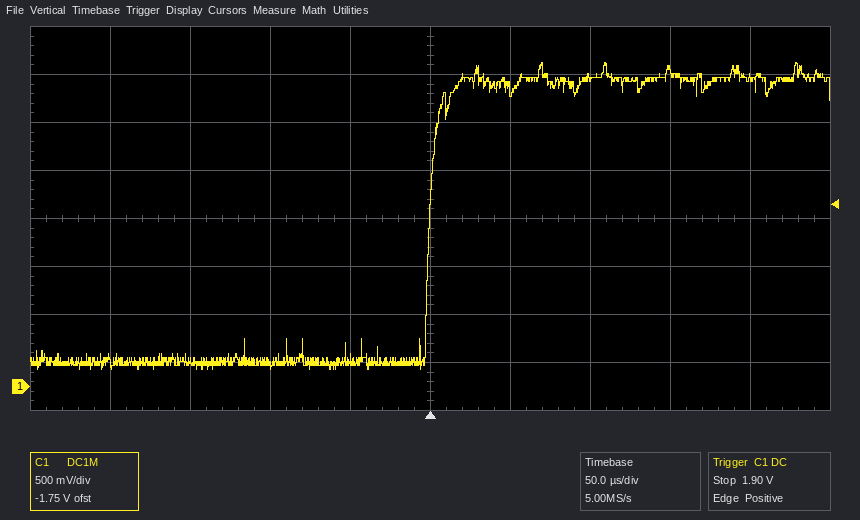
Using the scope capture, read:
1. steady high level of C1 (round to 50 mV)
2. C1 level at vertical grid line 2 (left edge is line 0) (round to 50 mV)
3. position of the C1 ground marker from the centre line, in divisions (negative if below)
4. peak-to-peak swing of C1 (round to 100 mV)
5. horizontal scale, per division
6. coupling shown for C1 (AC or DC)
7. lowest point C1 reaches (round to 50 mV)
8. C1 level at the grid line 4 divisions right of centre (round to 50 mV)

3.20 V
250 mV
-3.5 div
3.20 V
50 µs
DC
200 mV
3.20 V
